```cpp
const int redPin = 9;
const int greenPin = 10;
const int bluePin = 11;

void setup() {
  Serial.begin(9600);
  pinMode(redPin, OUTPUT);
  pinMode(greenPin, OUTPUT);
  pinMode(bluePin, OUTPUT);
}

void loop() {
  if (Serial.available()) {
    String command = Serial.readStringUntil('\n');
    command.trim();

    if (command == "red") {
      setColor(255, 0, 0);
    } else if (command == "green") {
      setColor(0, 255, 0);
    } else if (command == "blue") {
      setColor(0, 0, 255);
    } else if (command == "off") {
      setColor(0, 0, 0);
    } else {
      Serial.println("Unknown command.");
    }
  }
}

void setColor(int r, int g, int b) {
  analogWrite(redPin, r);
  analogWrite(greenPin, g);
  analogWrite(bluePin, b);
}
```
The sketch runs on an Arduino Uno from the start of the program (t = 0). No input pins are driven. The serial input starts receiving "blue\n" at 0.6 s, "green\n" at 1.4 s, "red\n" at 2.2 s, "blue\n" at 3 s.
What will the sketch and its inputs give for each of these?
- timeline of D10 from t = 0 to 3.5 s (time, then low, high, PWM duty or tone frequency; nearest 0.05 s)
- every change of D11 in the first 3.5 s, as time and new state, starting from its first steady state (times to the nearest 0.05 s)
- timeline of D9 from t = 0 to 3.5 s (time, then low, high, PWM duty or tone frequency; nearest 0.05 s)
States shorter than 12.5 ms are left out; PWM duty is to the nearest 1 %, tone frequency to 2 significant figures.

0 s low; 1.4 s high; 2.2 s low
0 s low; 0.6 s high; 1.4 s low; 3 s high
0 s low; 2.2 s high; 3 s low
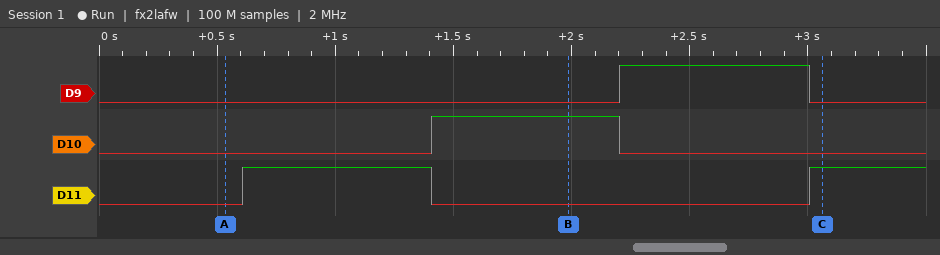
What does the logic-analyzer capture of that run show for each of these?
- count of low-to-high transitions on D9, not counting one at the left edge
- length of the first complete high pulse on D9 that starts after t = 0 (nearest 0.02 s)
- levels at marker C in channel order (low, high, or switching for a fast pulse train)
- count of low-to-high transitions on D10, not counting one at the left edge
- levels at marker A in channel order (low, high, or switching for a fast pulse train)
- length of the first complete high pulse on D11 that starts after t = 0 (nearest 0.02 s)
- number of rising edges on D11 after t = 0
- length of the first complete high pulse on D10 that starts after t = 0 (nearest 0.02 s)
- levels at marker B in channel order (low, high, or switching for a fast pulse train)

1
0.80 s
D9 low, D10 low, D11 high
1
D9 low, D10 low, D11 low
0.80 s
2
0.80 s
D9 low, D10 high, D11 low
